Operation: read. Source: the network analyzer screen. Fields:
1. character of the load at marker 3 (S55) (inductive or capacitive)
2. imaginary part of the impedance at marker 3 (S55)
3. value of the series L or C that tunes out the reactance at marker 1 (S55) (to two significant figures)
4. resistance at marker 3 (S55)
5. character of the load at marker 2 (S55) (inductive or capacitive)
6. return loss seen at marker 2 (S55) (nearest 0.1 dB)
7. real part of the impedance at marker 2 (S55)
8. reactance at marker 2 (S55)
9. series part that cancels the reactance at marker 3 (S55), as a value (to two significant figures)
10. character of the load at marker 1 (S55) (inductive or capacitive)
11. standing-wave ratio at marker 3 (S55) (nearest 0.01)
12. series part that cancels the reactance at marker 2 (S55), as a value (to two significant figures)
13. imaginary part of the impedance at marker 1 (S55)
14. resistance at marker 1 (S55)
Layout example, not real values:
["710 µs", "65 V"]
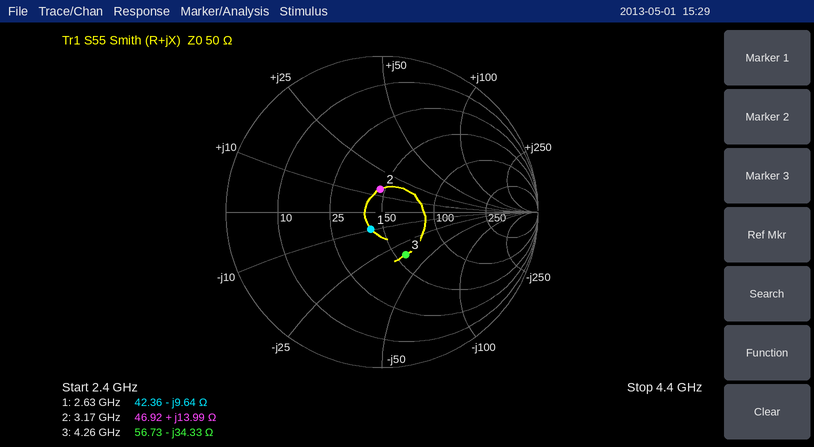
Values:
["capacitive", "-34.33 Ω", "580 pH", "56.73 Ω", "inductive", "16.7 dB", "46.92 Ω", "+13.99 Ω", "1.3 nH", "capacitive", "1.91", "3.6 pF", "-9.64 Ω", "42.36 Ω"]
